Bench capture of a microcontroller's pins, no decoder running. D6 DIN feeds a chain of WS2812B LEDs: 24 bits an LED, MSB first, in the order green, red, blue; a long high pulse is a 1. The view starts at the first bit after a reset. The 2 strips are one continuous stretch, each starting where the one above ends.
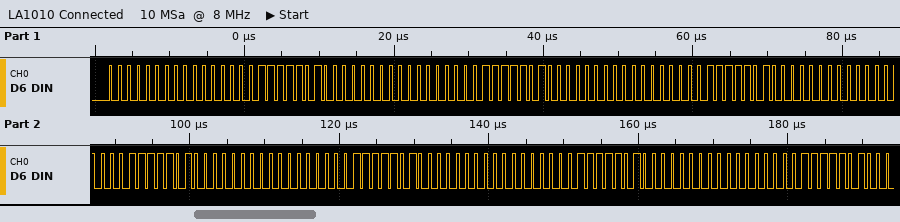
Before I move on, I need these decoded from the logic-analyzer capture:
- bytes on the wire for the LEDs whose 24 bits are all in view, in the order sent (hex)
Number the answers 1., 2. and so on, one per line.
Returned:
1. 00 00 FA 00 00 FA 00 00 FA 00 00 FA 00 00 FA 00 00 FA 00 00 FA
